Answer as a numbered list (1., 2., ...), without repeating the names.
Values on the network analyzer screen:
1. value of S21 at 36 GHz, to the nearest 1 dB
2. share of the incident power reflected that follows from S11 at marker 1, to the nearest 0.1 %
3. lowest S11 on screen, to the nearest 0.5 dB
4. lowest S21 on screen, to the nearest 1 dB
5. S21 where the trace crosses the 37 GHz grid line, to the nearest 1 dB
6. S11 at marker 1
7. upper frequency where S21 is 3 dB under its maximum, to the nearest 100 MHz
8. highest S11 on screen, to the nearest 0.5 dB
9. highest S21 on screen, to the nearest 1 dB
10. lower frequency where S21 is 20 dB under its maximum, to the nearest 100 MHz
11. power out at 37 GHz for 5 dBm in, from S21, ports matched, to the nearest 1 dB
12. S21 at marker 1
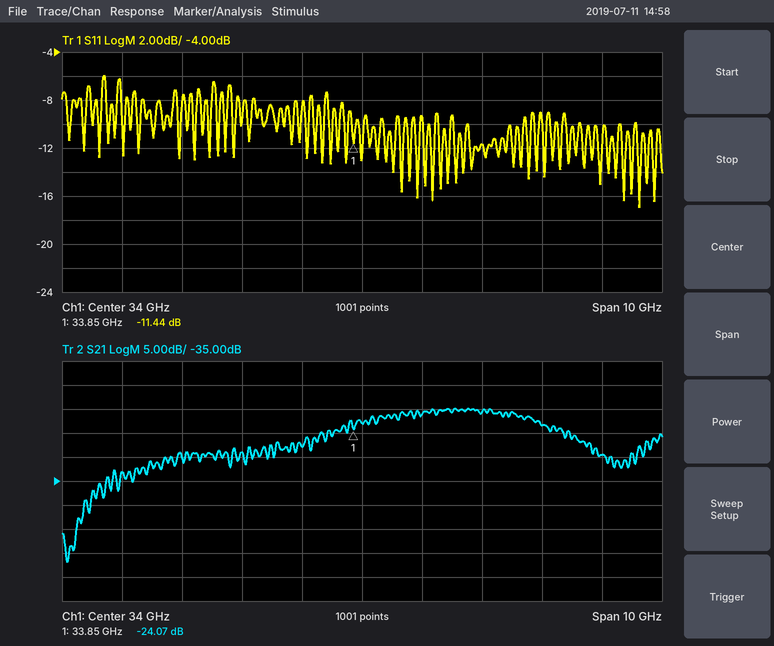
1. -21 dB
2. 7.2 %
3. -17.0 dB
4. -52 dB
5. -23 dB
6. -11.44 dB
7. 37.0 GHz
8. -6.0 dB
9. -20 dB
10. 29.5 GHz
11. -18 dBm
12. -24.07 dB
